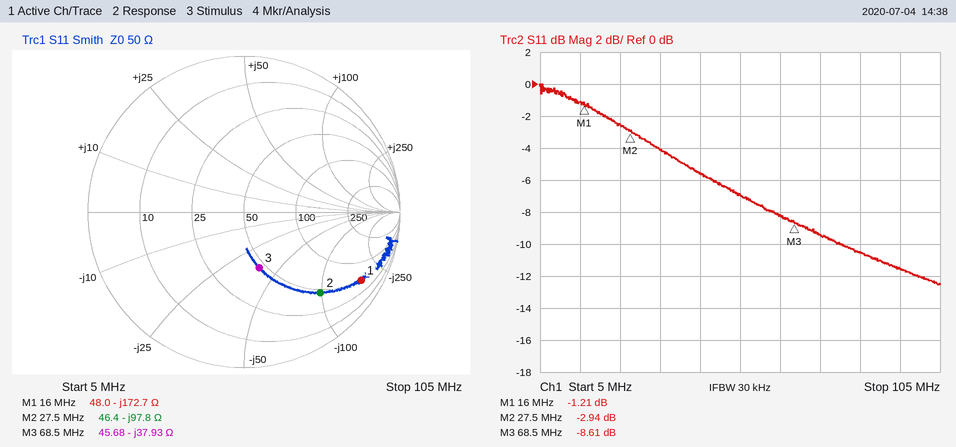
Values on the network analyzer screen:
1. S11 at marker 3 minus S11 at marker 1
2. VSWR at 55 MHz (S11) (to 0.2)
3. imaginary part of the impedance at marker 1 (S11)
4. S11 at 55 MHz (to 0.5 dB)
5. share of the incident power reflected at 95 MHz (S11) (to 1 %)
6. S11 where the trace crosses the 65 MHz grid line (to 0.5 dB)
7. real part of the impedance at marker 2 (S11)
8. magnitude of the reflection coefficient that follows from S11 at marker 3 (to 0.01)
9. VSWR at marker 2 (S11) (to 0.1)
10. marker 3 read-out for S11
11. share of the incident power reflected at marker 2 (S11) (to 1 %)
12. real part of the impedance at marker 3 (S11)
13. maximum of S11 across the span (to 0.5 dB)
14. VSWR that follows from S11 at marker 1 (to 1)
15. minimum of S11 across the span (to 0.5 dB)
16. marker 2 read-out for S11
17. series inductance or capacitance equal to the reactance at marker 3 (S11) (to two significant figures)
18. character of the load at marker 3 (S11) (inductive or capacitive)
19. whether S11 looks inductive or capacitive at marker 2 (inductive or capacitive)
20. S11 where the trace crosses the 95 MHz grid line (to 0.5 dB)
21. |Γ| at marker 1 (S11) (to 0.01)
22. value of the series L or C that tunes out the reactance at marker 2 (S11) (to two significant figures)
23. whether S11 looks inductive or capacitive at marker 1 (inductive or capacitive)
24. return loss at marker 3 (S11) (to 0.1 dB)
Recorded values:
-7.40 dB
2.6
-172.7 Ω
-7.0 dB
7 %
-8.0 dB
46.4 Ω
0.37
6.0
-8.61 dB
51 %
45.68 Ω
0.0 dB
14
-12.5 dB
-2.94 dB
61 pF
capacitive
capacitive
-11.5 dB
0.87
570 nH
capacitive
8.6 dB
